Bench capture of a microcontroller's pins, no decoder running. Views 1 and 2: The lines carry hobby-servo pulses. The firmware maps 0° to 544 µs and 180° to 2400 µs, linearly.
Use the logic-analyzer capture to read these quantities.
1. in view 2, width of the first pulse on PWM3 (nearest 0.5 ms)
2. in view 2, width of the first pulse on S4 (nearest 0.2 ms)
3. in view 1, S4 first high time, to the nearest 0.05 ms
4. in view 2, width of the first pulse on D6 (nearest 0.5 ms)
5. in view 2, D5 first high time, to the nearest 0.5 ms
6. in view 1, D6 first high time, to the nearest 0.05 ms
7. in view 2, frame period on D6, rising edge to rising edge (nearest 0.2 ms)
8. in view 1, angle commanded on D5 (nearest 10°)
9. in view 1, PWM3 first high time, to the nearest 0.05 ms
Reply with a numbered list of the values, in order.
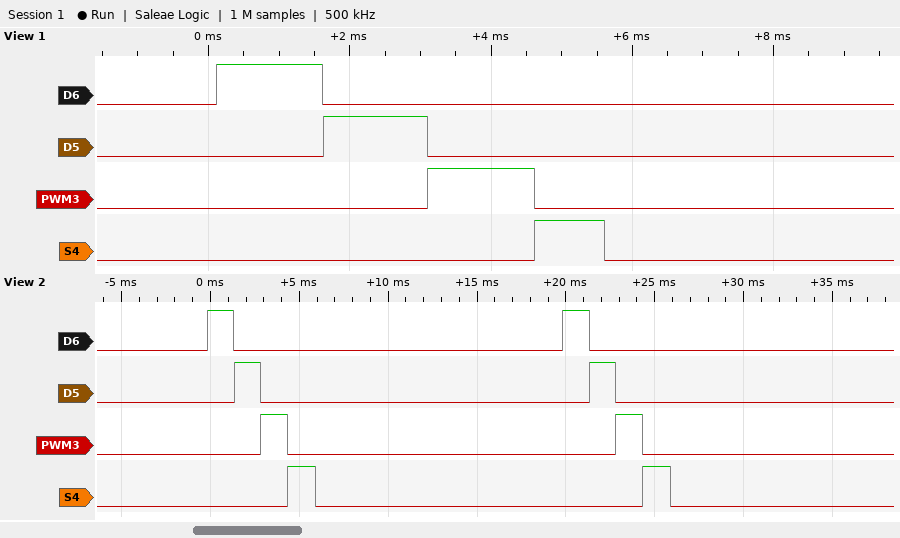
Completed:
1. 1.5 ms
2. 1.6 ms
3. 1.00 ms
4. 1.5 ms
5. 1.5 ms
6. 1.50 ms
7. 20.0 ms
8. 90°
9. 1.50 ms
